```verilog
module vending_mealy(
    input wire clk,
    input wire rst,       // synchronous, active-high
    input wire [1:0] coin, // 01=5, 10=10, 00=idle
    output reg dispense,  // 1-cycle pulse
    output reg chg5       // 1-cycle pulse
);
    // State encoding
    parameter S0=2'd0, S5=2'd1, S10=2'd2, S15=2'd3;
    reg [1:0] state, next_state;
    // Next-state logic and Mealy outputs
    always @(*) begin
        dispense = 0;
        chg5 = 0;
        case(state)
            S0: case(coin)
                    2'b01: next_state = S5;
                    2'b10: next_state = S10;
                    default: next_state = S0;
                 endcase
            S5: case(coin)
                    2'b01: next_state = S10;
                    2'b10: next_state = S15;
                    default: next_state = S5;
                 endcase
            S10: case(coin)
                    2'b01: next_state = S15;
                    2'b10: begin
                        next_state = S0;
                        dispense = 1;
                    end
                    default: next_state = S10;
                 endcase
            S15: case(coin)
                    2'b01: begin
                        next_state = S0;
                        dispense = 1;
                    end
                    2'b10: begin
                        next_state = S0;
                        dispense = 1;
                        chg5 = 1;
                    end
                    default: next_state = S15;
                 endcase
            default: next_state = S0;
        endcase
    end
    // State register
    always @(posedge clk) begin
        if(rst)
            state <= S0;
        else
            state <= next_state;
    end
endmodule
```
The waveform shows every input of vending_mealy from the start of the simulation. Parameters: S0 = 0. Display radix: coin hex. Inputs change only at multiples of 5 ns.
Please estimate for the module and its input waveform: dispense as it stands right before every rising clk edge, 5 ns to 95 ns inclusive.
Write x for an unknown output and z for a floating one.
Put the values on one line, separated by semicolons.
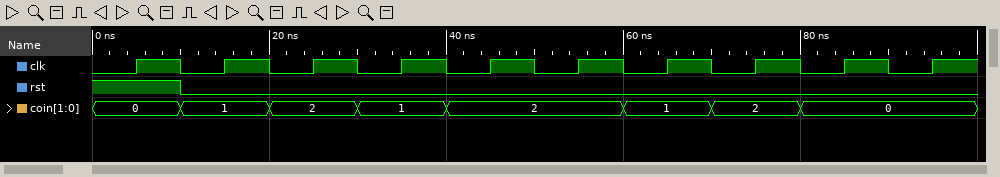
0 0 0 1 0 1 0 0 0 0
